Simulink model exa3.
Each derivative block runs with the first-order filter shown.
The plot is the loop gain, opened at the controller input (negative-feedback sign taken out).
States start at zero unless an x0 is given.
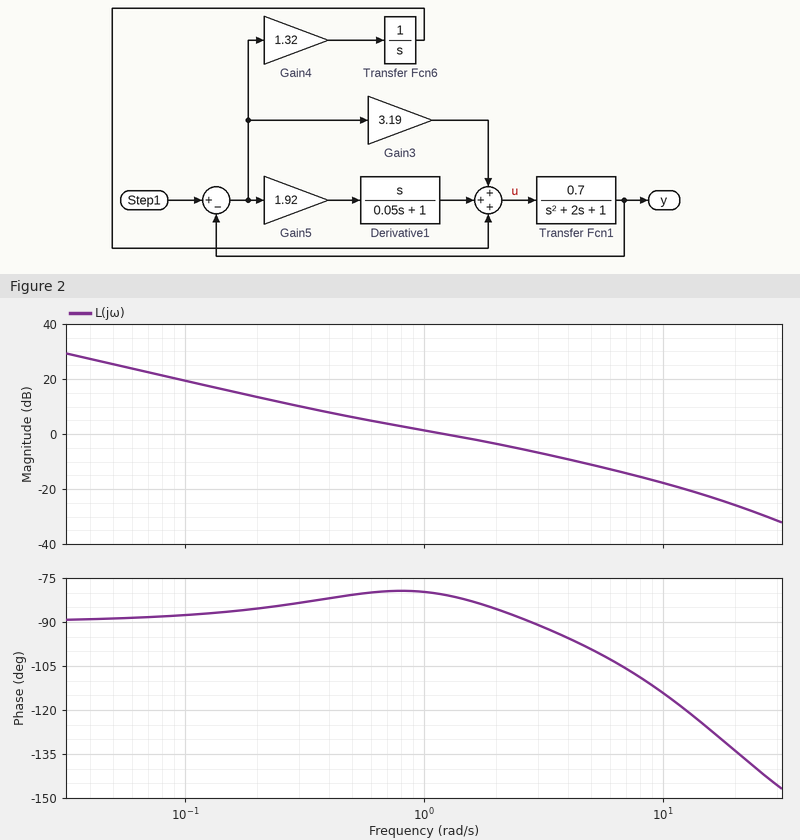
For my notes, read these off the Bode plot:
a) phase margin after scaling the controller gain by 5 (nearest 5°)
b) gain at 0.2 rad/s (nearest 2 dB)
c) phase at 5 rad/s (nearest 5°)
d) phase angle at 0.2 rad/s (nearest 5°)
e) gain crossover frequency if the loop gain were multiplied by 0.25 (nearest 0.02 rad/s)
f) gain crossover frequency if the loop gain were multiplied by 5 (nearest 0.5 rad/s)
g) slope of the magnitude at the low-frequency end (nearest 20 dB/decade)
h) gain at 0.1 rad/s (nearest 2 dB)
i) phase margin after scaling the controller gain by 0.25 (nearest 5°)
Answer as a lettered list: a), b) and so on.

a) 75°
b) 14 dB
c) -100°
d) -85°
e) 0.24 rad/s
f) 7.0 rad/s
g) -20 dB/decade
h) 20 dB
i) 95°
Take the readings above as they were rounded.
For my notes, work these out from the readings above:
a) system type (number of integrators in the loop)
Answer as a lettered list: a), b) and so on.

a) 1
